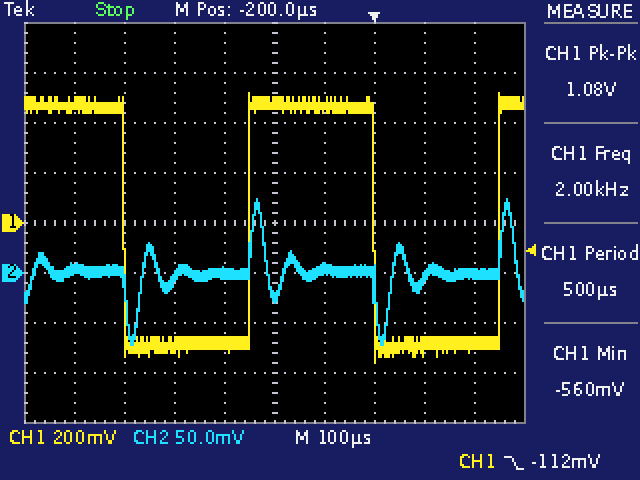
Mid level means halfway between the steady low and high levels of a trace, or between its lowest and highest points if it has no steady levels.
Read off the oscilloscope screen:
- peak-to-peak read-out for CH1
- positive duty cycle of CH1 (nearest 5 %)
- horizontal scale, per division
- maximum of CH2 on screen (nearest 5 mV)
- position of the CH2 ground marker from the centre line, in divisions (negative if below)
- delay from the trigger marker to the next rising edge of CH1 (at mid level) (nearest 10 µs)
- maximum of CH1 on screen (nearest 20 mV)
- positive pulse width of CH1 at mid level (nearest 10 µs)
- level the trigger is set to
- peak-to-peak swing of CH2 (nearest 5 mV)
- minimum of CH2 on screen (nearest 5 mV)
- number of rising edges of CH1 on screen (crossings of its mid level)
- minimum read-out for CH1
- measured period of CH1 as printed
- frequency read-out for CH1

1.08 V
50 %
100 µs
75 mV
-1.0 div
250 µs
520 mV
250 µs
-112 mV
145 mV
-70 mV
2
-560 mV
500 µs
2.00 kHz
